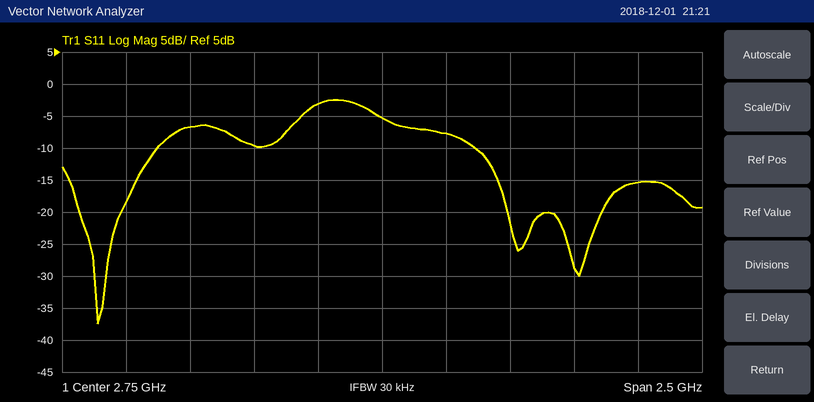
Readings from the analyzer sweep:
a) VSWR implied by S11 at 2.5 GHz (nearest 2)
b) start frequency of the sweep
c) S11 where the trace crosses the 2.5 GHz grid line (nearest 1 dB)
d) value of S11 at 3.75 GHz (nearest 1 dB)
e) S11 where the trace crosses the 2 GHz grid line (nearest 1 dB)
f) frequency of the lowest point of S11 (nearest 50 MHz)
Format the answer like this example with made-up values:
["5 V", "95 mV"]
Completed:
["6", "1.5 GHz", "-3 dB", "-15 dB", "-7 dB", "1.65 GHz"]
